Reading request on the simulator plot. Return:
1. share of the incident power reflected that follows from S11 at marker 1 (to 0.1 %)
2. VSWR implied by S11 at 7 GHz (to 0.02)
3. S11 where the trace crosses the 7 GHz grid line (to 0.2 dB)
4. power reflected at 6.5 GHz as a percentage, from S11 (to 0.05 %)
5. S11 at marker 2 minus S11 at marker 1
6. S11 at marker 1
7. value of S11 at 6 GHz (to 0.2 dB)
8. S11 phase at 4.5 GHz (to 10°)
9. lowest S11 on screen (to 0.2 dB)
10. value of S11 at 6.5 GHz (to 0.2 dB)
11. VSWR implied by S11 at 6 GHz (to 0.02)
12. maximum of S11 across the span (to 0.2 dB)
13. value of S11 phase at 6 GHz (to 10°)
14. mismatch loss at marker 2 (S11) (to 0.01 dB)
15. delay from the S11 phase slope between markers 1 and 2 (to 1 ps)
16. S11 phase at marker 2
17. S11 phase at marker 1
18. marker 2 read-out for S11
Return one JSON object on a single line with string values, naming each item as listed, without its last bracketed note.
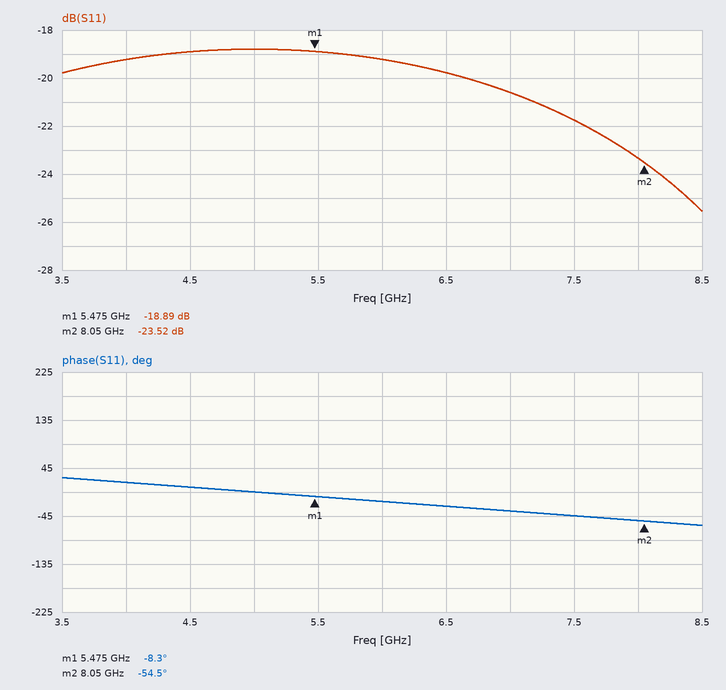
{"share of the incident power reflected that follows from S11 at marker 1": "1.3 %", "VSWR implied by S11 at 7 GHz": "1.20", "S11 where the trace crosses the 7 GHz grid line": "-20.6 dB", "power reflected at 6.5 GHz as a percentage, from S11": "1.05 %", "S11 at marker 2 minus S11 at marker 1": "-4.63 dB", "S11 at marker 1": "-18.89 dB", "value of S11 at 6 GHz": "-19.2 dB", "S11 phase at 4.5 GHz": "10°", "lowest S11 on screen": "-25.6 dB", "value of S11 at 6.5 GHz": "-19.8 dB", "VSWR implied by S11 at 6 GHz": "1.24", "maximum of S11 across the span": "-18.8 dB", "value of S11 phase at 6 GHz": "-20°", "mismatch loss at marker 2 (S11)": "0.02 dB", "delay from the S11 phase slope between markers 1 and 2": "50 ps", "S11 phase at marker 2": "-54.5°", "S11 phase at marker 1": "-8.3°", "marker 2 read-out for S11": "-23.52 dB"}
